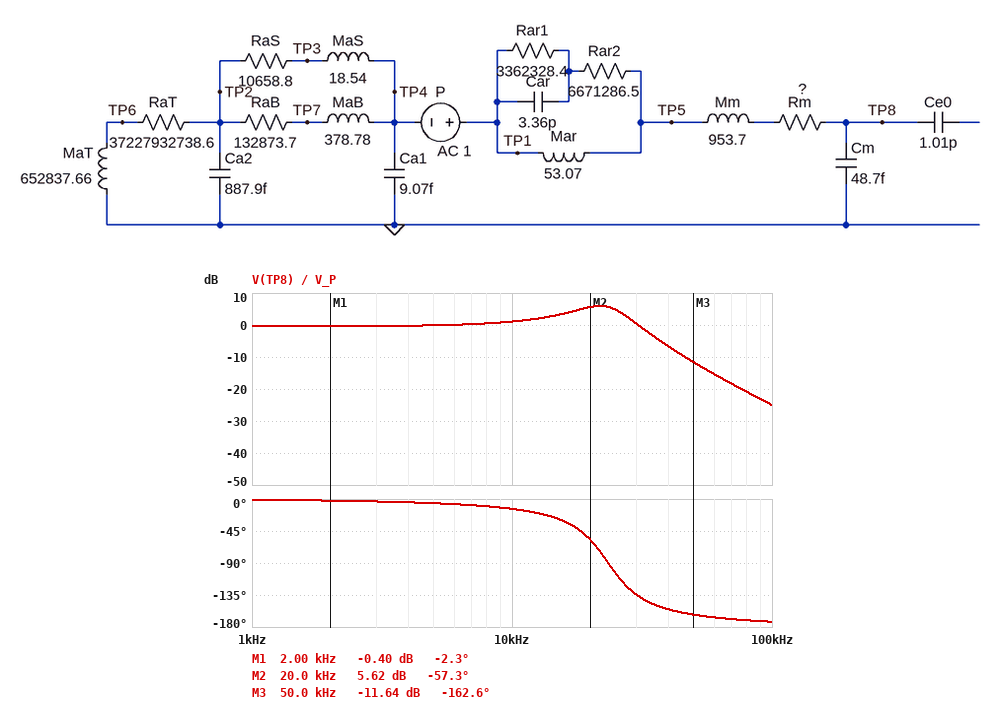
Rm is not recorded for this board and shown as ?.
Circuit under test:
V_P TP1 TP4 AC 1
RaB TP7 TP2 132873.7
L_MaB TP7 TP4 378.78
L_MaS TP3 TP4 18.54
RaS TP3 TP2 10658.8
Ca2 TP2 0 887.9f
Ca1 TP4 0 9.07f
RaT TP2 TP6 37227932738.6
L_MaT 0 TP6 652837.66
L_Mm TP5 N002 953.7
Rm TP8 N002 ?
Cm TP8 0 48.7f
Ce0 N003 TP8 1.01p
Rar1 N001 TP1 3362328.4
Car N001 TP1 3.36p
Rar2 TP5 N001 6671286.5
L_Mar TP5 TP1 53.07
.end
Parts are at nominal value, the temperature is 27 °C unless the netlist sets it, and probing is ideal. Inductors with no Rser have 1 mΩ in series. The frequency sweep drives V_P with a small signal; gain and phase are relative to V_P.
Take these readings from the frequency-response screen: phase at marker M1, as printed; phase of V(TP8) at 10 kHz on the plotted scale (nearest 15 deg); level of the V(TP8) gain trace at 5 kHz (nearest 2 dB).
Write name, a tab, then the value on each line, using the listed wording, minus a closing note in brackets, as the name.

phase at marker M1, as printed	-2.3 deg
phase of V(TP8) at 10 kHz on the plotted scale	-15 deg
level of the V(TP8) gain trace at 5 kHz	0 dB
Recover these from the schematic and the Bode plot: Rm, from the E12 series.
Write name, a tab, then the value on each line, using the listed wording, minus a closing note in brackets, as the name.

Rm, from the E12 series	68 MΩ
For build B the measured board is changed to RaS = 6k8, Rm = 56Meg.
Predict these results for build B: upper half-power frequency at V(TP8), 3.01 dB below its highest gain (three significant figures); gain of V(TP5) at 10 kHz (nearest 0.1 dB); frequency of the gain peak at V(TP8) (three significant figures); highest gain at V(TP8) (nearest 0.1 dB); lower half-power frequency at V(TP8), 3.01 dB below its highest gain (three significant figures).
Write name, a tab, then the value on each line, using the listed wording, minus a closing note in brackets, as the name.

upper half-power frequency at V(TP8), 3.01 dB below its highest gain	26.9 kHz
gain of V(TP5) at 10 kHz	-0.4 dB
frequency of the gain peak at V(TP8)	22.3 kHz
highest gain at V(TP8)	7.4 dB
lower half-power frequency at V(TP8), 3.01 dB below its highest gain	16.6 kHz
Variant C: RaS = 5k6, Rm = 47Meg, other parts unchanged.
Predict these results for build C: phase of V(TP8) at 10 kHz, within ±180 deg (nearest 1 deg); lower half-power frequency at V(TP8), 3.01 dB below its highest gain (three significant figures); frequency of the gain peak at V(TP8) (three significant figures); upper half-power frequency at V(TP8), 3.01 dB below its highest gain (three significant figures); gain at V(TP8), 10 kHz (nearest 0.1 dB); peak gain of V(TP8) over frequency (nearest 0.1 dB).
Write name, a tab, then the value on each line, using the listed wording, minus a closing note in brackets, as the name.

phase of V(TP8) at 10 kHz, within ±180 deg	-10 deg
lower half-power frequency at V(TP8), 3.01 dB below its highest gain	17.9 kHz
frequency of the gain peak at V(TP8)	22.6 kHz
upper half-power frequency at V(TP8), 3.01 dB below its highest gain	26.6 kHz
gain at V(TP8), 10 kHz	1.2 dB
peak gain of V(TP8) over frequency	8.8 dB
